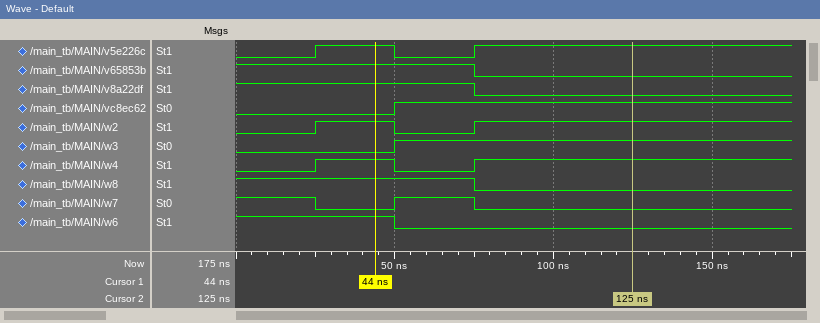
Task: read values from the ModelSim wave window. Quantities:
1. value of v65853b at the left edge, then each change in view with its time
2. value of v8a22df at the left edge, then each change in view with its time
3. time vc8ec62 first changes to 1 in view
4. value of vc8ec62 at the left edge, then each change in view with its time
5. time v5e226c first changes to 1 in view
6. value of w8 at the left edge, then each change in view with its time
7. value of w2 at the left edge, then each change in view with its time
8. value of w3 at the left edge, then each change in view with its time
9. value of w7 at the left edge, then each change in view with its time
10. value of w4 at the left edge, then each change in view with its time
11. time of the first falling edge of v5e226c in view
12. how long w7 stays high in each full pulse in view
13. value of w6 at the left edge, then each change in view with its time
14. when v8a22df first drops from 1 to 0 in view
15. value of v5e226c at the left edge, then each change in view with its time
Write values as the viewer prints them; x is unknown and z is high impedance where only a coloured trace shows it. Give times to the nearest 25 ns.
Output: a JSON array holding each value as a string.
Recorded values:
["1, 0 at 75 ns", "1, 0 at 75 ns", "50 ns", "0, 1 at 50 ns", "25 ns", "1, 0 at 75 ns", "0, 1 at 25 ns, 0 at 50 ns, 1 at 75 ns", "0, 1 at 50 ns", "1, 0 at 25 ns, 1 at 50 ns, 0 at 75 ns", "0, 1 at 25 ns, 0 at 50 ns, 1 at 75 ns", "50 ns", "25 ns", "1, 0 at 50 ns", "75 ns", "0, 1 at 25 ns, 0 at 50 ns, 1 at 75 ns"]
